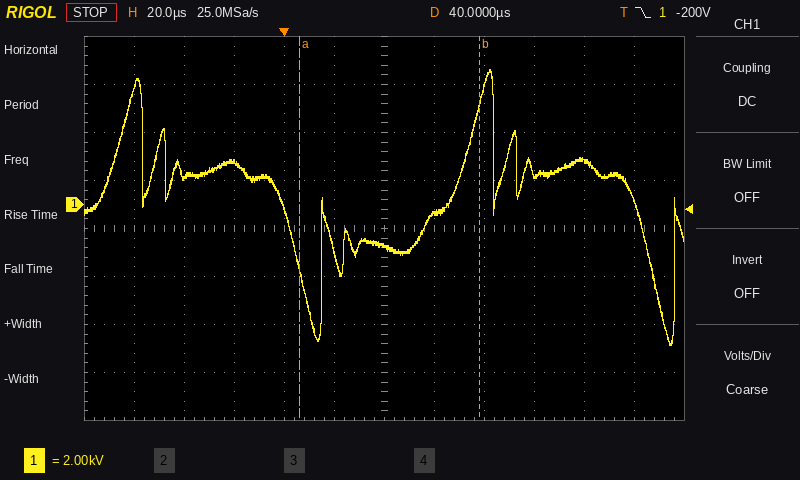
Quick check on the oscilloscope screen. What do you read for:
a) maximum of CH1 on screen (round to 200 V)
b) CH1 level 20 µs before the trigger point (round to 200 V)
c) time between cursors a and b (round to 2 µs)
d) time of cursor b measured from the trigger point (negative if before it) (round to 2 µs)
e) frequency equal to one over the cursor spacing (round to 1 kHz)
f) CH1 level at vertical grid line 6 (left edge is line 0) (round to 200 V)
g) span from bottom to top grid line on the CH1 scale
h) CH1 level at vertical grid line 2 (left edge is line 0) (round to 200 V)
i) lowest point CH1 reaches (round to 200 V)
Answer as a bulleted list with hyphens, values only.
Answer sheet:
- 5.6 kV
- 1.8 kV
- 72 µs
- +78 µs
- 14 kHz
- -1.8 kV
- 16 kV
- 1.2 kV
- -5.8 kV
